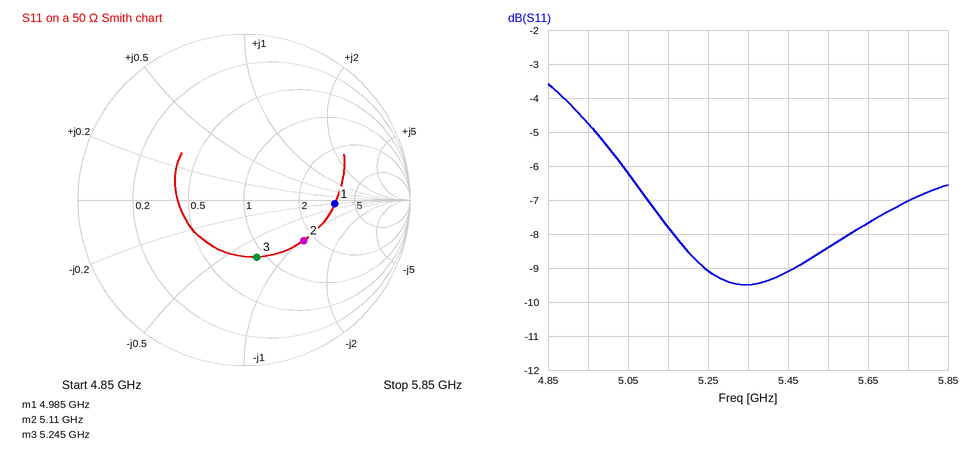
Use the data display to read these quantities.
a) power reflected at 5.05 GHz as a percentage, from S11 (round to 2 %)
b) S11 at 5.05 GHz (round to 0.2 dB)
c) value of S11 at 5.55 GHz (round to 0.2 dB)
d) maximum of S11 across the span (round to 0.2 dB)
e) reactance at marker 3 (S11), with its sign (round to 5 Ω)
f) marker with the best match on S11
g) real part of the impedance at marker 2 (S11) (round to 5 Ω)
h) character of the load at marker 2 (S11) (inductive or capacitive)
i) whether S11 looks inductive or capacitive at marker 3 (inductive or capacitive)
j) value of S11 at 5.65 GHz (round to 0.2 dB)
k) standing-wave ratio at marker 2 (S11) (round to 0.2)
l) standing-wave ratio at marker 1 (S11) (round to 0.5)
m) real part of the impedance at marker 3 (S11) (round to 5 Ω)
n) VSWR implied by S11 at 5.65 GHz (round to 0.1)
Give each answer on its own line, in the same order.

24 %
-6.2 dB
-8.4 dB
-3.6 dB
-35 Ω
marker 3
85 Ω
capacitive
capacitive
-7.6 dB
2.6
3.5
45 Ω
2.4
